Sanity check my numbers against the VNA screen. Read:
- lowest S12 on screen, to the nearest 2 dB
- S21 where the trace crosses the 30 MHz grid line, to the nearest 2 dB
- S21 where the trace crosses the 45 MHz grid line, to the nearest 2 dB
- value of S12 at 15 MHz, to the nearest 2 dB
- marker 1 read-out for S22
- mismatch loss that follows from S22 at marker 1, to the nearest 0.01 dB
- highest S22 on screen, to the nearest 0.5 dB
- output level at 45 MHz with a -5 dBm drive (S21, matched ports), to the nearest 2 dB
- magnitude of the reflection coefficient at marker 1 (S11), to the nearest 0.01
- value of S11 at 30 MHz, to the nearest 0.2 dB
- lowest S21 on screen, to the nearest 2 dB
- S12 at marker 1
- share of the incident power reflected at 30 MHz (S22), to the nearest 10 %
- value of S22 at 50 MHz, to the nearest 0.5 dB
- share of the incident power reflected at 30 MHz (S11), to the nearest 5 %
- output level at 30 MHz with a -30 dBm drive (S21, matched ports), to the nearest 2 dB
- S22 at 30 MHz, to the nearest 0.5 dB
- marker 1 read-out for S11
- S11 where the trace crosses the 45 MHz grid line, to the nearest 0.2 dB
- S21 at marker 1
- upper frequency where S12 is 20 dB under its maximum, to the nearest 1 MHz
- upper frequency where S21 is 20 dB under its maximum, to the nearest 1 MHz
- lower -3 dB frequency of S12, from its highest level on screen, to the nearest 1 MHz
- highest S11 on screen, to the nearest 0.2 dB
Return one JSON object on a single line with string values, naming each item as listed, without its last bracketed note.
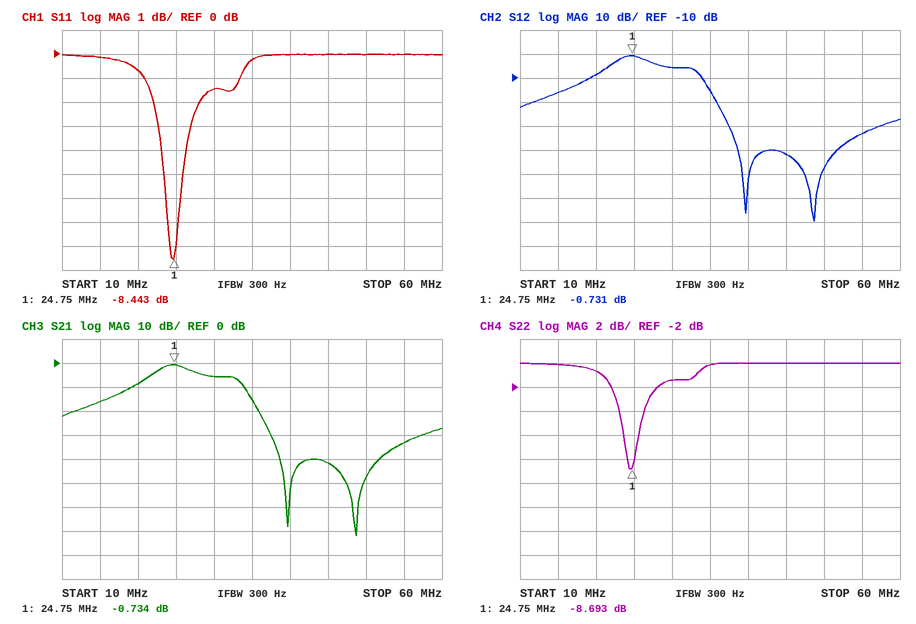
{"lowest S12 on screen, to the nearest 2 dB": "-70 dB", "S21 where the trace crosses the 30 MHz grid line, to the nearest 2 dB": "-6 dB", "S21 where the trace crosses the 45 MHz grid line, to the nearest 2 dB": "-42 dB", "value of S12 at 15 MHz, to the nearest 2 dB": "-16 dB", "marker 1 read-out for S22": "-8.693 dB", "mismatch loss that follows from S22 at marker 1, to the nearest 0.01 dB": "0.63 dB", "highest S22 on screen, to the nearest 0.5 dB": "0.0 dB", "output level at 45 MHz with a -5 dBm drive (S21, matched ports), to the nearest 2 dB": "-46 dBm", "magnitude of the reflection coefficient at marker 1 (S11), to the nearest 0.01": "0.38", "value of S11 at 30 MHz, to the nearest 0.2 dB": "-1.4 dB", "lowest S21 on screen, to the nearest 2 dB": "-72 dB", "S12 at marker 1": "-0.731 dB", "share of the incident power reflected at 30 MHz (S22), to the nearest 10 %": "70 %", "value of S22 at 50 MHz, to the nearest 0.5 dB": "0.0 dB", "share of the incident power reflected at 30 MHz (S11), to the nearest 5 %": "70 %", "output level at 30 MHz with a -30 dBm drive (S21, matched ports), to the nearest 2 dB": "-36 dBm", "S22 at 30 MHz, to the nearest 0.5 dB": "-1.5 dB", "marker 1 read-out for S11": "-8.443 dB", "S11 where the trace crosses the 45 MHz grid line, to the nearest 0.2 dB": "0.0 dB", "S21 at marker 1": "-0.734 dB", "upper frequency where S12 is 20 dB under its maximum, to the nearest 1 MHz": "36 MHz", "upper frequency where S21 is 20 dB under its maximum, to the nearest 1 MHz": "36 MHz", "lower -3 dB frequency of S12, from its highest level on screen, to the nearest 1 MHz": "22 MHz", "highest S11 on screen, to the nearest 0.2 dB": "0.0 dB"}
